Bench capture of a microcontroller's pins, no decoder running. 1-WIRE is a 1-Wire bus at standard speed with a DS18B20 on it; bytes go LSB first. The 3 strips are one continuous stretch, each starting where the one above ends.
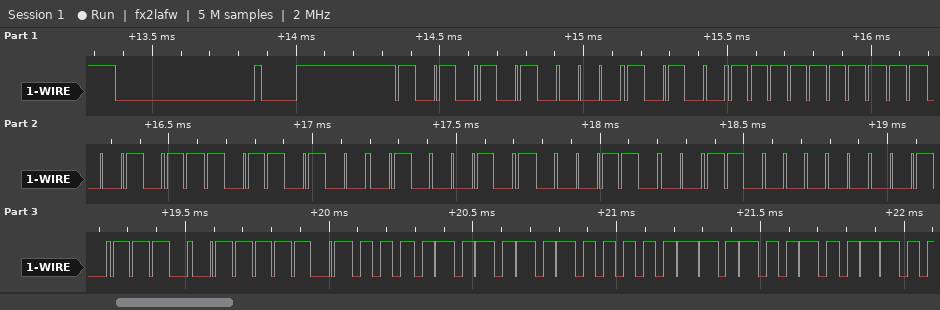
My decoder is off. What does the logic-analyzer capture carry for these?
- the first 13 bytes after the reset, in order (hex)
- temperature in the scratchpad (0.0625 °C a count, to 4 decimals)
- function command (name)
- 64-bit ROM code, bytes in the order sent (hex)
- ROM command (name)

55 28 FF D3 2D A2 18 03 74 BE 50 05 4B
85.0000 °C
Read Scratchpad
28 FF D3 2D A2 18 03 74
Match ROM
